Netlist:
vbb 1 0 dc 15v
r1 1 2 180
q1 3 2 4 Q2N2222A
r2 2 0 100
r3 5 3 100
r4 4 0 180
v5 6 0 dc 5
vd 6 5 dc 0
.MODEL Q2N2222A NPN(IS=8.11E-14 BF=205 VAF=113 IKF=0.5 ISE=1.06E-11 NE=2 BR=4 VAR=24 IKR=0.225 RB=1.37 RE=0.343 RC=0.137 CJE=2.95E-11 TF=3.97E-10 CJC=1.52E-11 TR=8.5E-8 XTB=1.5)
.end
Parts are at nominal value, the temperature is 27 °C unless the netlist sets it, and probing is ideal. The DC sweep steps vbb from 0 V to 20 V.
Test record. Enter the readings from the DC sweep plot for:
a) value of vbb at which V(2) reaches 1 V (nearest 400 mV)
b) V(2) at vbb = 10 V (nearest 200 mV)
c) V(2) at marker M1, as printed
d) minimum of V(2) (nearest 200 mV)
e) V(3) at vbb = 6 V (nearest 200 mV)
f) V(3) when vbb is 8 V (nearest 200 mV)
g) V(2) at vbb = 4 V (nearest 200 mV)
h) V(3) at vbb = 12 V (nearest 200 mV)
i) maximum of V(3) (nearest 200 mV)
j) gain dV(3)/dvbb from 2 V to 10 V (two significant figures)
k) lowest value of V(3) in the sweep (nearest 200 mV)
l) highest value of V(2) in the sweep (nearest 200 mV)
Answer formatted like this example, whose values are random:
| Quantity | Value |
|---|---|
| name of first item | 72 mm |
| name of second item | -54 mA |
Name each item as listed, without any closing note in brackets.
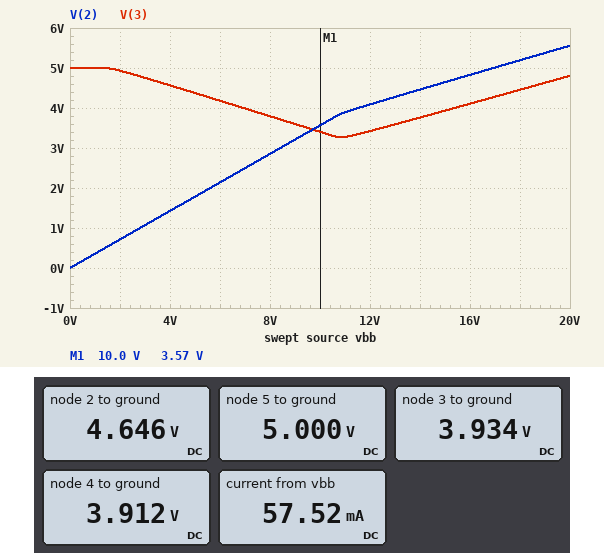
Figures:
| Quantity | Value |
|---|---|
| value of vbb at which V(2) reaches 1 V | 2.8 V |
| V(2) at vbb = 10 V | 3.6 V |
| V(2) at marker M1, as printed | 3.57 V |
| minimum of V(2) | 0 V |
| V(3) at vbb = 6 V | 4.2 V |
| V(3) when vbb is 8 V | 3.8 V |
| V(2) at vbb = 4 V | 1.4 V |
| V(3) at vbb = 12 V | 3.4 V |
| maximum of V(3) | 5.0 V |
| gain dV(3)/dvbb from 2 V to 10 V | -0.19 V/V |
| lowest value of V(3) in the sweep | 3.2 V |
| highest value of V(2) in the sweep | 5.6 V |
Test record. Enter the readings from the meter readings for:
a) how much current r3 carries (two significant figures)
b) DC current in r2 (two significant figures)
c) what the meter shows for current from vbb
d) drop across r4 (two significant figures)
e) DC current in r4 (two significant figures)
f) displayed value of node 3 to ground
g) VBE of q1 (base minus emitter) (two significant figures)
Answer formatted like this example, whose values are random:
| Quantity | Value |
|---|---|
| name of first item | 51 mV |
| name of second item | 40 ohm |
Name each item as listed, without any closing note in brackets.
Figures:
| Quantity | Value |
|---|---|
| how much current r3 carries | 11 mA |
| DC current in r2 | 46 mA |
| what the meter shows for current from vbb | 57.52 mA |
| drop across r4 | 3.9 V |
| DC current in r4 | 22 mA |
| displayed value of node 3 to ground | 3.934 V |
| VBE of q1 (base minus emitter) | 730 mV |
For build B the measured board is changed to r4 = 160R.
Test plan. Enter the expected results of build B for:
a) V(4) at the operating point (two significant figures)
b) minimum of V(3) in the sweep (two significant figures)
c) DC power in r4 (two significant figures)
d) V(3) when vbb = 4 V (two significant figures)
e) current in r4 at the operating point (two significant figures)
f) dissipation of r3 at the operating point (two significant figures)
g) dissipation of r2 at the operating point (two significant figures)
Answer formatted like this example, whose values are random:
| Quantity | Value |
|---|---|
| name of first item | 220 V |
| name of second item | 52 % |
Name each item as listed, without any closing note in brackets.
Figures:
| Quantity | Value |
|---|---|
| V(4) at the operating point | 3.8 V |
| minimum of V(3) in the sweep | 3.1 V |
| DC power in r4 | 91 mW |
| V(3) when vbb = 4 V | 4.5 V |
| current in r4 at the operating point | 24 mA |
| dissipation of r3 at the operating point | 13 mW |
| dissipation of r2 at the operating point | 210 mW |
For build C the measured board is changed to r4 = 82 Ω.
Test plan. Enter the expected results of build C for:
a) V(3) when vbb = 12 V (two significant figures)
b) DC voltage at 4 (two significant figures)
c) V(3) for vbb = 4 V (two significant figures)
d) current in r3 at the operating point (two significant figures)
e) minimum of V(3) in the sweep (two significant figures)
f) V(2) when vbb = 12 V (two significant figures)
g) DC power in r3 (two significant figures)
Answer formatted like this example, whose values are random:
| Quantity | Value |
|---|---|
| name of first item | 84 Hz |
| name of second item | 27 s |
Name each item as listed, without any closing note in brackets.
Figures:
| Quantity | Value |
|---|---|
| V(3) when vbb = 12 V | 2.8 V |
| DC voltage at 4 | 3.2 V |
| V(3) for vbb = 4 V | 4.1 V |
| current in r3 at the operating point | 18 mA |
| minimum of V(3) in the sweep | 2.3 V |
| V(2) when vbb = 12 V | 3.5 V |
| DC power in r3 | 31 mW |
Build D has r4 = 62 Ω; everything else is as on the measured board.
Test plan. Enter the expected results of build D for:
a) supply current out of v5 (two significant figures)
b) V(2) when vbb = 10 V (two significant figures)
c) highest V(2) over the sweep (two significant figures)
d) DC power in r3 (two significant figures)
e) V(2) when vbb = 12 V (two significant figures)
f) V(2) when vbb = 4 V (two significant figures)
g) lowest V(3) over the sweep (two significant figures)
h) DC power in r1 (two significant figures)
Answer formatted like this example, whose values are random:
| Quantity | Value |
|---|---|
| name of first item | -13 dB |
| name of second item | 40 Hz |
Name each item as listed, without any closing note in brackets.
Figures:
| Quantity | Value |
|---|---|
| supply current out of v5 | 21 mA |
| V(2) when vbb = 10 V | 3.0 V |
| highest V(2) over the sweep | 4.4 V |
| DC power in r3 | 43 mW |
| V(2) when vbb = 12 V | 3.3 V |
| V(2) when vbb = 4 V | 1.4 V |
| lowest V(3) over the sweep | 2.0 V |
| DC power in r1 | 710 mW |
